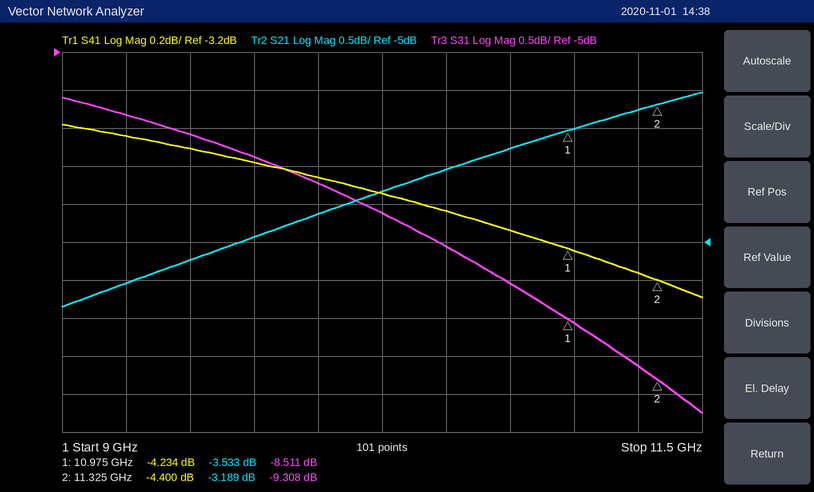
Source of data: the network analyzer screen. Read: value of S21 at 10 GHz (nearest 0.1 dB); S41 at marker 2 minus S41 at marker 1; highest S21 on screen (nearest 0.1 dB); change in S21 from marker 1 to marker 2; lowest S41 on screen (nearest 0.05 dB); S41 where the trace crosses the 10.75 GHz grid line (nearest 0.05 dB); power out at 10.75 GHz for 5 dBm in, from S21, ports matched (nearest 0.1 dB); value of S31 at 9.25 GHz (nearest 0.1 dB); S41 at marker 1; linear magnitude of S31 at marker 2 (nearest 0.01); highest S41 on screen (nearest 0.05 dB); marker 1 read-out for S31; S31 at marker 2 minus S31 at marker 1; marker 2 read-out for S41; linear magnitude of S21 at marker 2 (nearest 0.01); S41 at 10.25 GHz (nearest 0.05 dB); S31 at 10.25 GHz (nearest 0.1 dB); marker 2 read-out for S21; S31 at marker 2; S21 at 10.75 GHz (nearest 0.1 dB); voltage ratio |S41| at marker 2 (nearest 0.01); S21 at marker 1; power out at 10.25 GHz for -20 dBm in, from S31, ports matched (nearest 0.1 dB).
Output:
-4.6 dB
-0.166 dB
-3.0 dB
0.344 dB
-4.50 dB
-4.15 dB
1.2 dBm
-5.8 dB
-4.234 dB
0.34
-3.60 dB
-8.511 dB
-0.797 dB
-4.400 dB
0.69
-3.95 dB
-7.1 dB
-3.189 dB
-9.308 dB
-3.8 dB
0.60
-3.533 dB
-27.1 dBm
